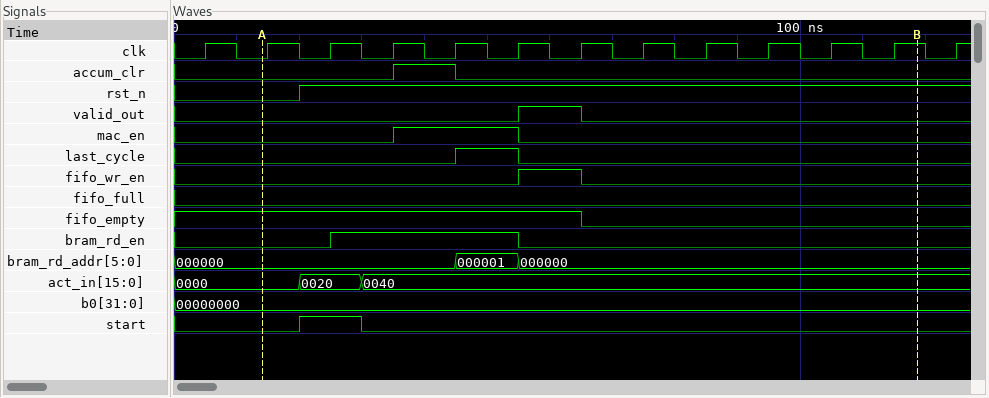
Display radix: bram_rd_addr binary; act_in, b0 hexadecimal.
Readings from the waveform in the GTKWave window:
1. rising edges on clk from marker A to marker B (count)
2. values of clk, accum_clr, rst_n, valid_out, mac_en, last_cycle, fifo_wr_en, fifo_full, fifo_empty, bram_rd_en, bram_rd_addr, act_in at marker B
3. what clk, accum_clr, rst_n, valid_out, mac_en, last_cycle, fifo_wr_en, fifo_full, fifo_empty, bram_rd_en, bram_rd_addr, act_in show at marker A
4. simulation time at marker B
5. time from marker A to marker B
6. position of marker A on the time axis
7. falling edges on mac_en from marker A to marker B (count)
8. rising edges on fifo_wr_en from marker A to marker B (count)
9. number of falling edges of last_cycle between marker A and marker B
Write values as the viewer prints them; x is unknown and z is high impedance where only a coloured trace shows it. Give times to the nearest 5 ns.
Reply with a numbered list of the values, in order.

1. 11
2. clk=1, accum_clr=0, rst_n=1, valid_out=0, mac_en=0, last_cycle=0, fifo_wr_en=0, fifo_full=0, fifo_empty=0, bram_rd_en=0, bram_rd_addr=000000, act_in=0040
3. clk=0, accum_clr=0, rst_n=0, valid_out=0, mac_en=0, last_cycle=0, fifo_wr_en=0, fifo_full=0, fifo_empty=1, bram_rd_en=0, bram_rd_addr=000000, act_in=0000
4. 120 ns
5. 105 ns
6. 15 ns
7. 1
8. 1
9. 1
